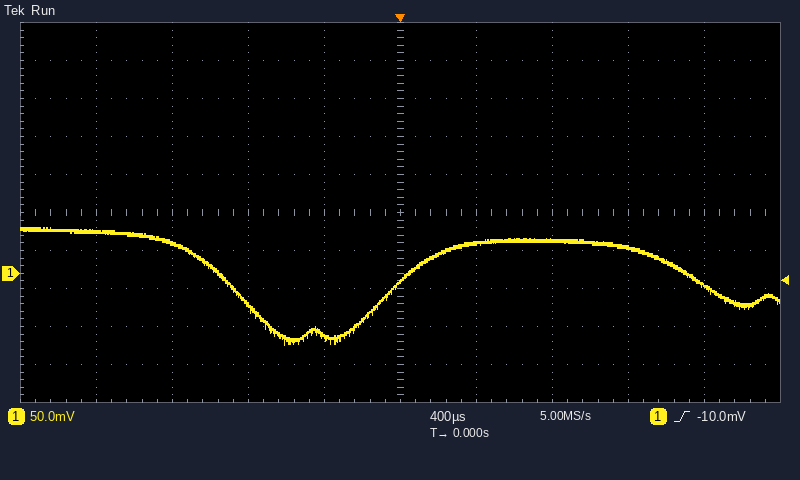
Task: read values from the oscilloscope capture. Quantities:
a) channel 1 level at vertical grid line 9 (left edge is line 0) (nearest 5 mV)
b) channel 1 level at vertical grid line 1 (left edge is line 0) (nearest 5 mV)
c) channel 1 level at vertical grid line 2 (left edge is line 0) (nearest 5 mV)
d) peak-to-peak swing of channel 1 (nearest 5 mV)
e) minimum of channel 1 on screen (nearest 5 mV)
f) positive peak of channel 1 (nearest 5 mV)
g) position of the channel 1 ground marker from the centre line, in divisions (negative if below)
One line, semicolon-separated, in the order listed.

-15 mV; 55 mV; 40 mV; 155 mV; -95 mV; 60 mV; -1.6 div
